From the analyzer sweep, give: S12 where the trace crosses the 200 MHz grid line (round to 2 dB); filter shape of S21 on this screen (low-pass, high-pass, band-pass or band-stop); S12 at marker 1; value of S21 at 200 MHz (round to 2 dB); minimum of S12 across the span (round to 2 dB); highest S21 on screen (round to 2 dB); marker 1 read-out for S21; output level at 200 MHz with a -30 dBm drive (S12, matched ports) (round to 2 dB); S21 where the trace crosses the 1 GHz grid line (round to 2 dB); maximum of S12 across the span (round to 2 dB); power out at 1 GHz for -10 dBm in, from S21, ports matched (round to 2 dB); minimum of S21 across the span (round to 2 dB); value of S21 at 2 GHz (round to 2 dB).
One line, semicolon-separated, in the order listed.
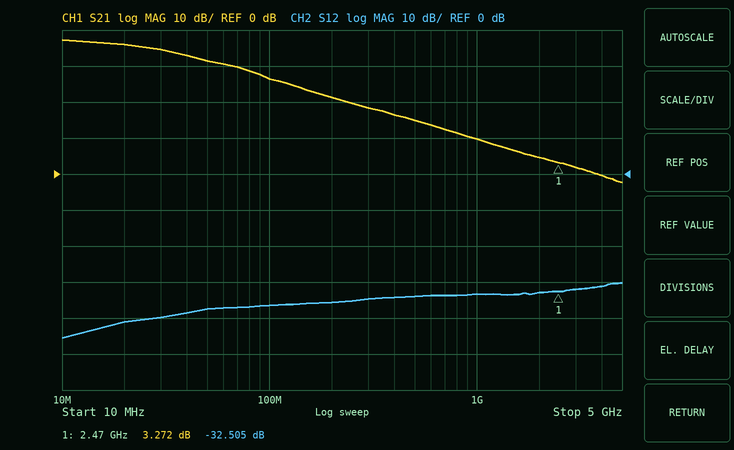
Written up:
-36 dB; low-pass; -32.505 dB; 22 dB; -46 dB; 38 dB; 3.272 dB; -66 dBm; 10 dB; -30 dB; 0 dBm; -2 dB; 4 dB
